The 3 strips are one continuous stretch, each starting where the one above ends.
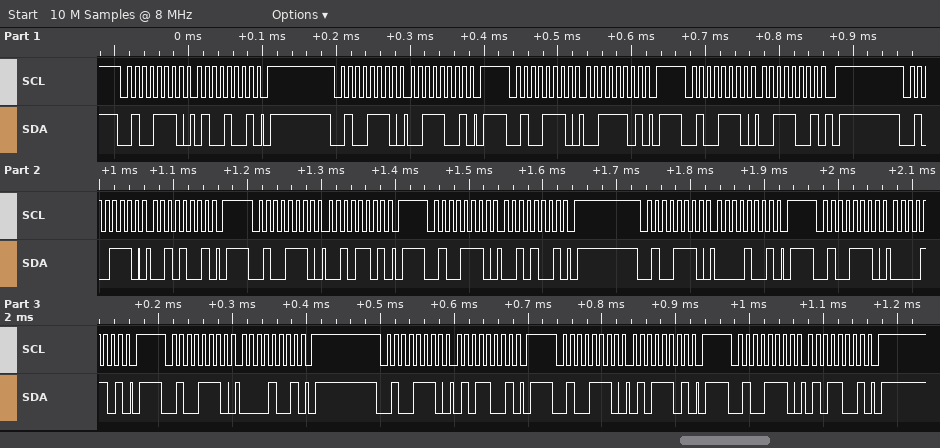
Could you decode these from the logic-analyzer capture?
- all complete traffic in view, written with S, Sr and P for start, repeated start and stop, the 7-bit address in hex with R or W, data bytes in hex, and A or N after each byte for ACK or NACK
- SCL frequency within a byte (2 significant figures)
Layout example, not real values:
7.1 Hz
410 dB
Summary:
S 27W A 49 A P S 27W A 39 A P S 27W A 3D A P S 27W A 39 A P S 27W A 29 A P S 27W A 2D A P S 27W A 29 A P S 27W A 09 A P S 27W A 0D A P S 27W A 09 A P S 27W A 59 A P S 27W A 5D A P S 27W A 59 A P
100 kHz
